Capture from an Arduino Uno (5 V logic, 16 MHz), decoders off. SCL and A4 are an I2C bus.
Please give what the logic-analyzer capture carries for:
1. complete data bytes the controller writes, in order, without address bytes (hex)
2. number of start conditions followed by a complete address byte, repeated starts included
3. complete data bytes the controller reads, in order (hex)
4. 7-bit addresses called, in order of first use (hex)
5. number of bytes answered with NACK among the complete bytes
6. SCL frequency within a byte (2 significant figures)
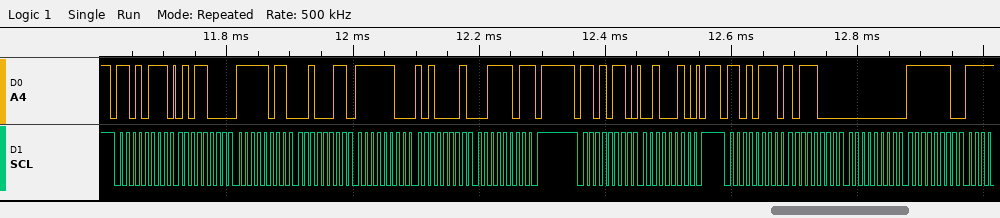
22
3
58 FB 23 FC A1 3D B8 00 FE
0x6B
1
100 kHz
